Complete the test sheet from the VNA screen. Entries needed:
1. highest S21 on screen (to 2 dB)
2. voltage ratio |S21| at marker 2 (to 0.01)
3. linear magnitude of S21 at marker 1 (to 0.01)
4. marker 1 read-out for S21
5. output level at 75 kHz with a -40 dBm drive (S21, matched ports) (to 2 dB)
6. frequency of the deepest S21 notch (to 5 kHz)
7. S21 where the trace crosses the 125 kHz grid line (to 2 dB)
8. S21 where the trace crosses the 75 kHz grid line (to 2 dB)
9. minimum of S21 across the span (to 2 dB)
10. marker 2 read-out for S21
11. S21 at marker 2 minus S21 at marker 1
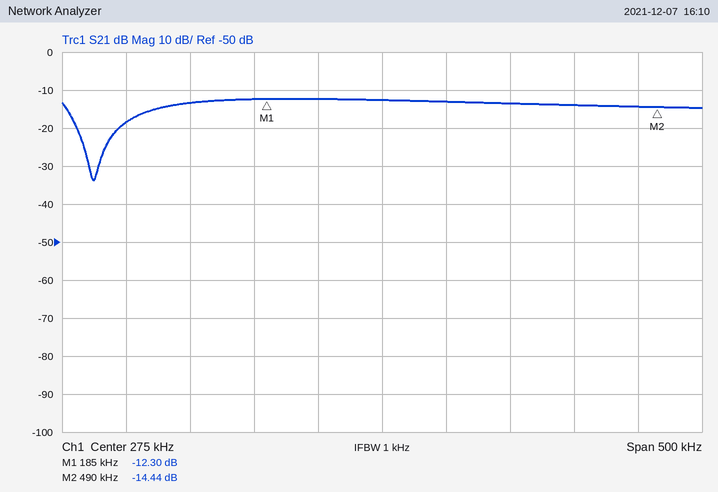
-12 dB
0.19
0.24
-12.30 dB
-58 dBm
50 kHz
-14 dB
-18 dB
-34 dB
-14.44 dB
-2.14 dB
